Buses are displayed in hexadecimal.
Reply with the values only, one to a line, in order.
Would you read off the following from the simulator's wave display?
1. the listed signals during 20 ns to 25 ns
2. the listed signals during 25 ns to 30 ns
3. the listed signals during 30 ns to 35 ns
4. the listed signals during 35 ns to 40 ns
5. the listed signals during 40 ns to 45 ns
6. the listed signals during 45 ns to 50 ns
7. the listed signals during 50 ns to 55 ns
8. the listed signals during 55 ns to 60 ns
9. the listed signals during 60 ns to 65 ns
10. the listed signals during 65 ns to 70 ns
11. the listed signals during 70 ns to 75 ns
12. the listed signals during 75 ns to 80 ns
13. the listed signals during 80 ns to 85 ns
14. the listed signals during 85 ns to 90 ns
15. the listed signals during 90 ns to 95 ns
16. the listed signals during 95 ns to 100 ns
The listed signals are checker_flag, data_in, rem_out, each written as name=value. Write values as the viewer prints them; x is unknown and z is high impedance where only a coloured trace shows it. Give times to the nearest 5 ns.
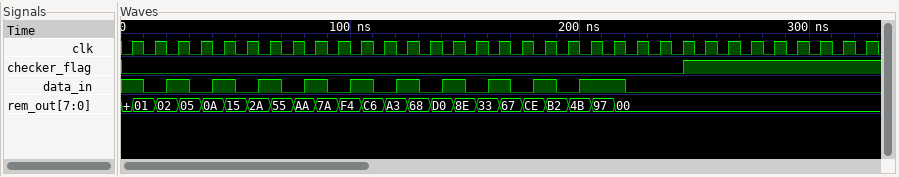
checker_flag=0, data_in=1, rem_out=02
checker_flag=0, data_in=1, rem_out=05
checker_flag=0, data_in=0, rem_out=05
checker_flag=0, data_in=0, rem_out=0A
checker_flag=0, data_in=1, rem_out=0A
checker_flag=0, data_in=1, rem_out=15
checker_flag=0, data_in=0, rem_out=15
checker_flag=0, data_in=0, rem_out=2A
checker_flag=0, data_in=1, rem_out=2A
checker_flag=0, data_in=1, rem_out=55
checker_flag=0, data_in=0, rem_out=55
checker_flag=0, data_in=0, rem_out=AA
checker_flag=0, data_in=1, rem_out=AA
checker_flag=0, data_in=1, rem_out=7A
checker_flag=0, data_in=0, rem_out=7A
checker_flag=0, data_in=0, rem_out=F4
